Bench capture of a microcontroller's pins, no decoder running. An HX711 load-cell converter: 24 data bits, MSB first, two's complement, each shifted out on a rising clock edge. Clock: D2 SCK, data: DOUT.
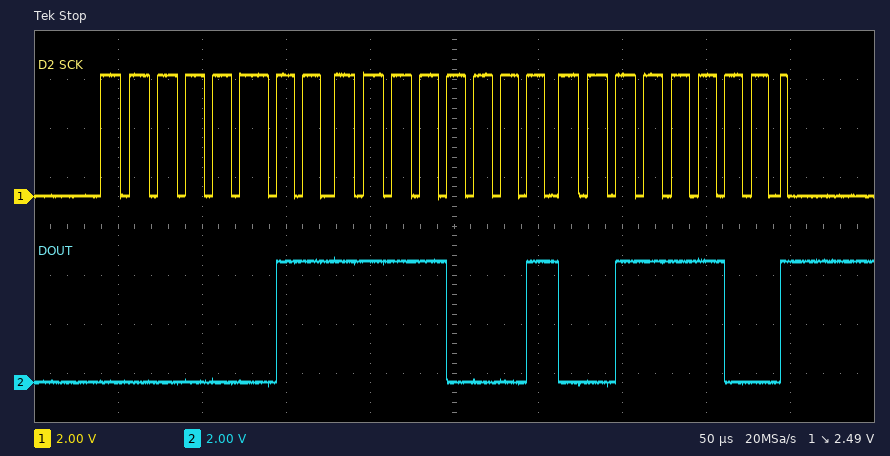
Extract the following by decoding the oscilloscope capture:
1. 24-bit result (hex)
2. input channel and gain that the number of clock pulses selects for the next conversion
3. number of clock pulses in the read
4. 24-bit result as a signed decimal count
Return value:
0x03F13C
channel A, gain 128
25
258364
